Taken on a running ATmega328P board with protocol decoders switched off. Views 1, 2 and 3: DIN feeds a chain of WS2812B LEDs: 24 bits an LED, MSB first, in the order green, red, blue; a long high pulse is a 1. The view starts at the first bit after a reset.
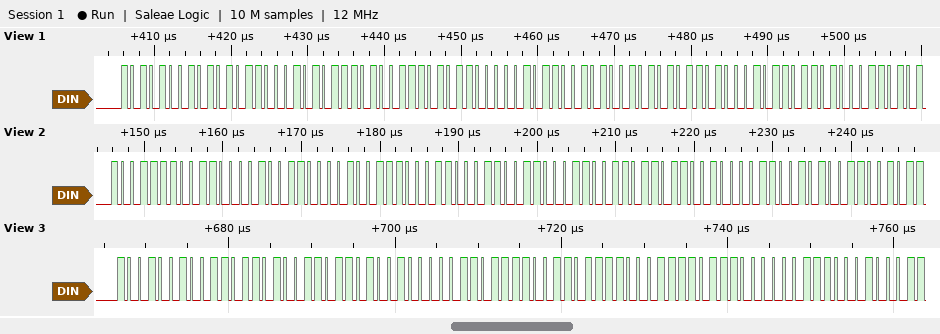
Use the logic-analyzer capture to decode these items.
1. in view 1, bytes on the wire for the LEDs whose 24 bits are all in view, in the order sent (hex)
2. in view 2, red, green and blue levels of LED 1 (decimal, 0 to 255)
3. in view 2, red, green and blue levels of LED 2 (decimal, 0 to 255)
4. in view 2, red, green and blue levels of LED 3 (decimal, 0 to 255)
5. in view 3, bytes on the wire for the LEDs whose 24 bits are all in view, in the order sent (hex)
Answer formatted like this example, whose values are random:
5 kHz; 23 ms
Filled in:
A9 56 2B A7 58 2C A5 5A 2D; 97, 158, 48; 99, 156, 49; 100, 155, 50; 92 6D 36 90 6F 37 8F 70 38
